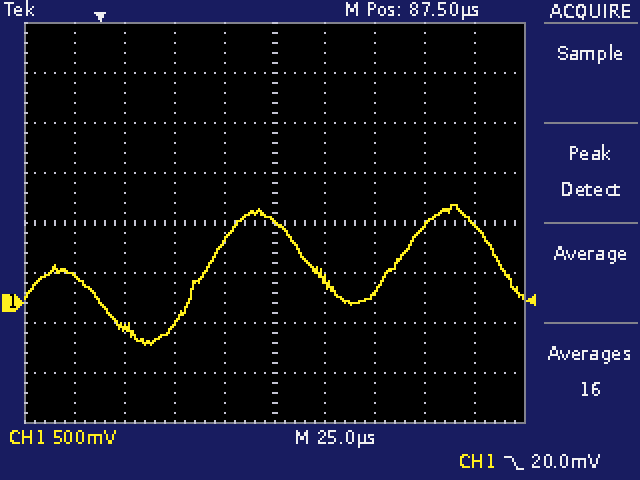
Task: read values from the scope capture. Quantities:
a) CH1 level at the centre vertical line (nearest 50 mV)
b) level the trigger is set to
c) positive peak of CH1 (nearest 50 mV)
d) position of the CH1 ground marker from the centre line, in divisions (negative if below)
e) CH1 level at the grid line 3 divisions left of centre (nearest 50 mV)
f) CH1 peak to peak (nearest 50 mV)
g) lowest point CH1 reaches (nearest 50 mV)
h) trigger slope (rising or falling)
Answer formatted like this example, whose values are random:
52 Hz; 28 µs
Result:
800 mV; 20.0 mV; 1.00 V; -1.6 div; -250 mV; 1.40 V; -400 mV; falling
